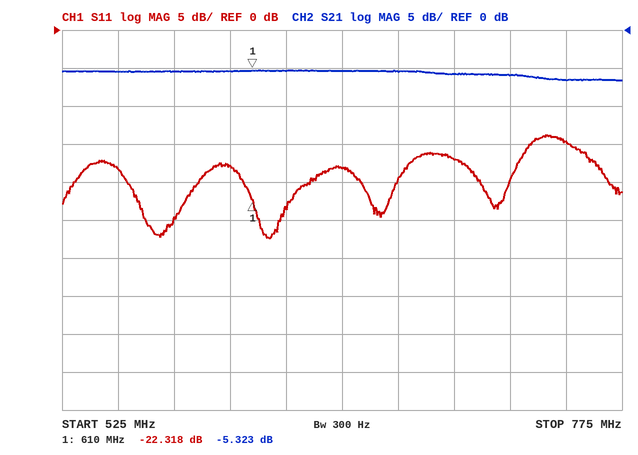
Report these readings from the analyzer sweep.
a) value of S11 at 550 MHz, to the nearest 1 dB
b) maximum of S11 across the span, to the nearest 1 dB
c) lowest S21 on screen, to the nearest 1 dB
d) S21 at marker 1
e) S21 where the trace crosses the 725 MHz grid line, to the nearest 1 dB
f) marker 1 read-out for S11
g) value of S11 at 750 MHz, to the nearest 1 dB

-18 dB
-14 dB
-7 dB
-5.323 dB
-6 dB
-22.318 dB
-15 dB
